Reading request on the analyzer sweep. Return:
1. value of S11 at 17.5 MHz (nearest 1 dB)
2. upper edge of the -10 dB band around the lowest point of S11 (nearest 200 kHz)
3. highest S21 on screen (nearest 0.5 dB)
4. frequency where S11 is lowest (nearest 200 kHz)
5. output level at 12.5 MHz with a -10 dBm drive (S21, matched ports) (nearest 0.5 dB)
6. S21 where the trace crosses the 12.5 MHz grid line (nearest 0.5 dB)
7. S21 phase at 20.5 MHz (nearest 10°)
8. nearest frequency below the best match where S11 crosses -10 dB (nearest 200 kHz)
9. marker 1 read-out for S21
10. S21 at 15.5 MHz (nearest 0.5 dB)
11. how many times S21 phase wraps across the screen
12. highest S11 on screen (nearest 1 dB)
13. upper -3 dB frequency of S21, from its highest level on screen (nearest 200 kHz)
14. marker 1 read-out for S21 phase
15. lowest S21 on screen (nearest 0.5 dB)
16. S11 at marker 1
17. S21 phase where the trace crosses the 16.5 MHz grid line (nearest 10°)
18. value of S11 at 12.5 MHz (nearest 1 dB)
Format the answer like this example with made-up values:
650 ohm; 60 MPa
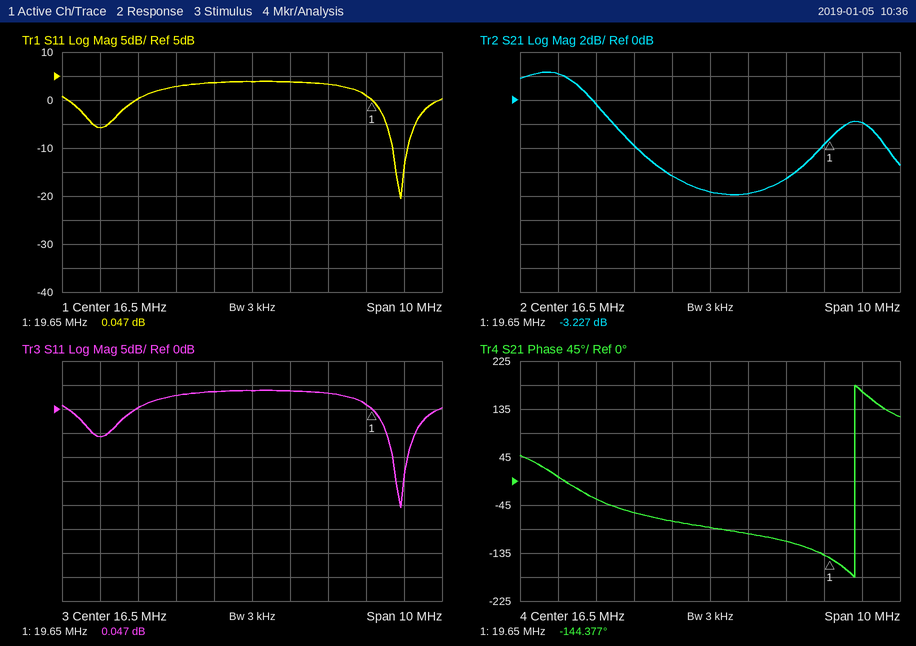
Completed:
4 dB; 20.6 MHz; 2.5 dB; 20.4 MHz; -8.0 dBm; 2.0 dB; 170°; 20.2 MHz; -3.227 dB; -6.5 dB; 1; 4 dB; 13.6 MHz; -144.377°; -8.0 dB; 0.047 dB; -90°; -6 dB
